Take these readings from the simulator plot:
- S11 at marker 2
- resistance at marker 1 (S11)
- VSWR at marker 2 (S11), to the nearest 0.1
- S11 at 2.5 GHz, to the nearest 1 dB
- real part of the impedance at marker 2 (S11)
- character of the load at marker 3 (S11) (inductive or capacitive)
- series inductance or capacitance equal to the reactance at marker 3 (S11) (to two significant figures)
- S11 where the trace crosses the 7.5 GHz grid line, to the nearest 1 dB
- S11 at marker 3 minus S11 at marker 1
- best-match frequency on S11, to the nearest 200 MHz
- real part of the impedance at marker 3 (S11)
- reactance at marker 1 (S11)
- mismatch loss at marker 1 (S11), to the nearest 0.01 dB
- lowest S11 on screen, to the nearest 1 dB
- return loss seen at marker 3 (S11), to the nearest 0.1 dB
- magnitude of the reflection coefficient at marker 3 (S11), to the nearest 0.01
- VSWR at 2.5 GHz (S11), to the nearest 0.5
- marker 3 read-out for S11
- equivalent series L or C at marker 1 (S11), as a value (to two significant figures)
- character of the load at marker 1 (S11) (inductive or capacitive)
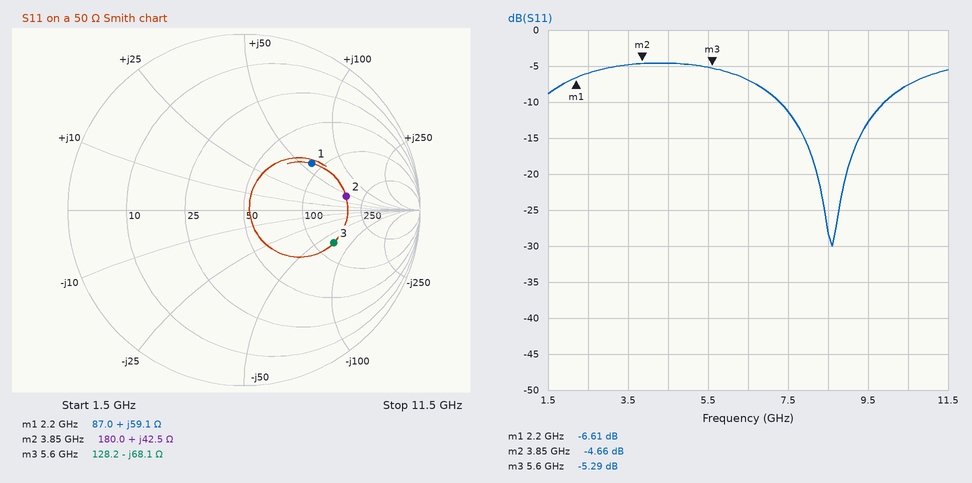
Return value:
-4.66 dB
87.0 Ω
3.8
-6 dB
180.0 Ω
capacitive
420 fF
-11 dB
1.32 dB
8.6 GHz
128.2 Ω
+59.1 Ω
1.07 dB
-30 dB
5.3 dB
0.54
3.0
-5.29 dB
4.3 nH
inductive
